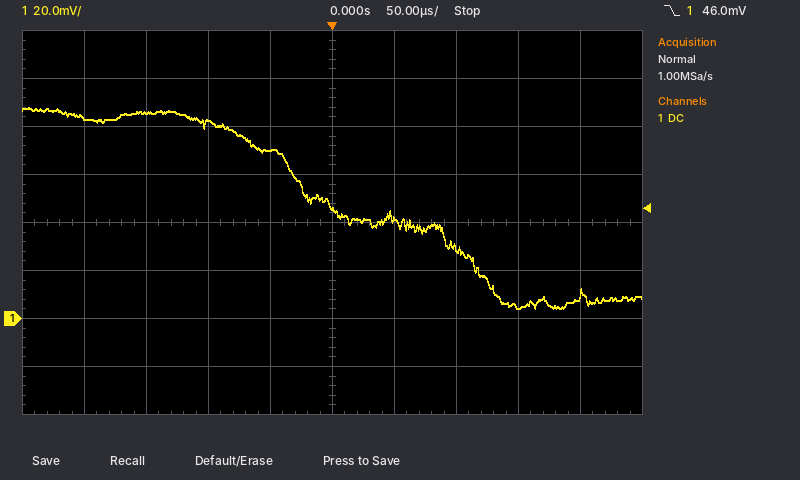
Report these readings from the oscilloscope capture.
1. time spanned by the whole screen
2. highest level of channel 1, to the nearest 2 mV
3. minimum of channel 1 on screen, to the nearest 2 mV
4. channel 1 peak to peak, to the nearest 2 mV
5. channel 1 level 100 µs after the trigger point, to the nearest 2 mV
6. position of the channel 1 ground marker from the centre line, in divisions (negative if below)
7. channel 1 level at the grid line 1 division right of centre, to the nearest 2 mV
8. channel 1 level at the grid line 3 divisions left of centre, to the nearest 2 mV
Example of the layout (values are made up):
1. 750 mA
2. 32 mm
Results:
1. 500 µs
2. 88 mV
3. 4 mV
4. 84 mV
5. 30 mV
6. -2.0 div
7. 42 mV
8. 86 mV
